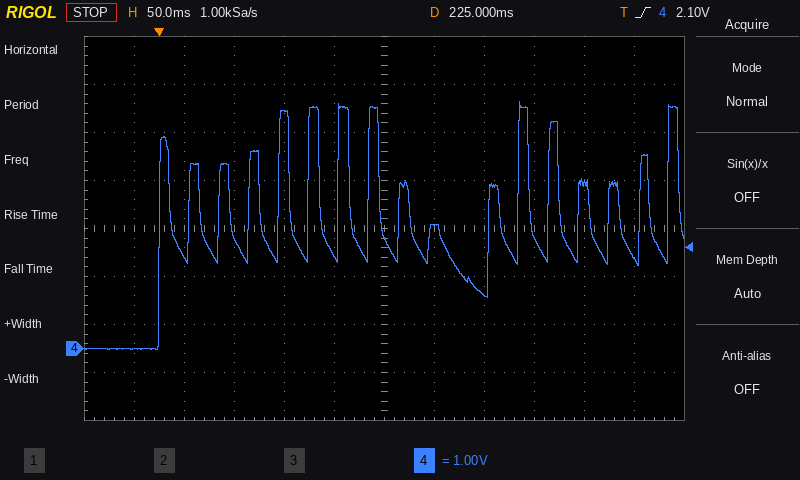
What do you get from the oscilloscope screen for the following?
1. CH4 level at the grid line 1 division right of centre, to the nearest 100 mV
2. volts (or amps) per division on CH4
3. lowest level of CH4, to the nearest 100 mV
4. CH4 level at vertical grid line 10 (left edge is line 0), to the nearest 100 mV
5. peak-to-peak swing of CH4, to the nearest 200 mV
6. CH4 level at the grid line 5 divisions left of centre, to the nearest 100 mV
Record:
2.6 V
1 V
0.0 V
3.5 V
5.2 V
0.0 V
